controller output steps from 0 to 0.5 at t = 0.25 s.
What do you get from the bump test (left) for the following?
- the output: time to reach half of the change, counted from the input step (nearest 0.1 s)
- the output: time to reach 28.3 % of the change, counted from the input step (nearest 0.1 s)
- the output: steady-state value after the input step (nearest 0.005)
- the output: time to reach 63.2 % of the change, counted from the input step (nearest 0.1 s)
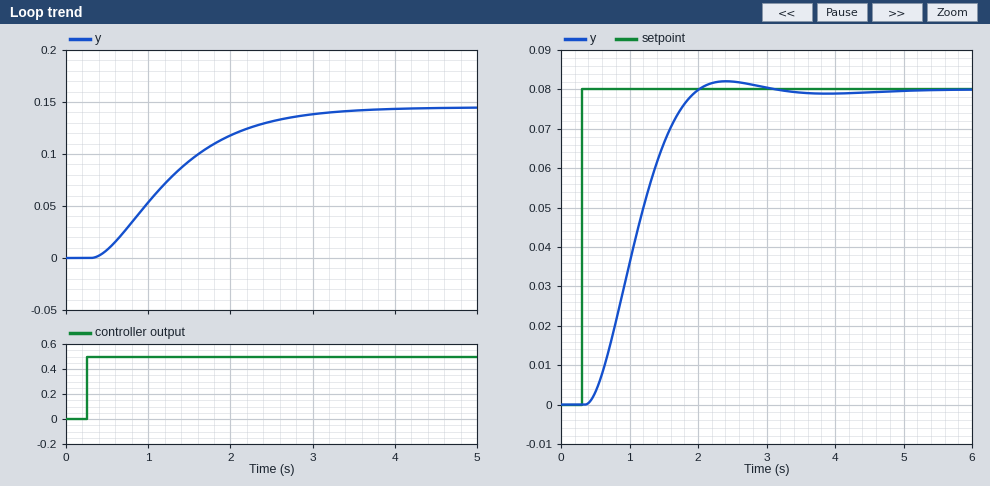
1.0 s
0.6 s
0.145
1.2 s
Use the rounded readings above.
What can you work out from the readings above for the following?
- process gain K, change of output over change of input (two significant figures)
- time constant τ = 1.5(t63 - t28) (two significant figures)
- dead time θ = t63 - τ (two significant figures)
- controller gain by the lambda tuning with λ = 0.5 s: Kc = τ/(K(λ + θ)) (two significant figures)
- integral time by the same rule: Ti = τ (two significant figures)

0.29
0.90 s
0.30 s
3.9
0.90 s
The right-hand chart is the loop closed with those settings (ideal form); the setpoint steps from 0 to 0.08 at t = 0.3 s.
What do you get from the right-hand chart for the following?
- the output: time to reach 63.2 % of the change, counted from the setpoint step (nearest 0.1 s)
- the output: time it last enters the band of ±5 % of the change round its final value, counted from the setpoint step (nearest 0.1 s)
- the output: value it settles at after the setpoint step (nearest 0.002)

0.9 s
1.5 s
0.080
